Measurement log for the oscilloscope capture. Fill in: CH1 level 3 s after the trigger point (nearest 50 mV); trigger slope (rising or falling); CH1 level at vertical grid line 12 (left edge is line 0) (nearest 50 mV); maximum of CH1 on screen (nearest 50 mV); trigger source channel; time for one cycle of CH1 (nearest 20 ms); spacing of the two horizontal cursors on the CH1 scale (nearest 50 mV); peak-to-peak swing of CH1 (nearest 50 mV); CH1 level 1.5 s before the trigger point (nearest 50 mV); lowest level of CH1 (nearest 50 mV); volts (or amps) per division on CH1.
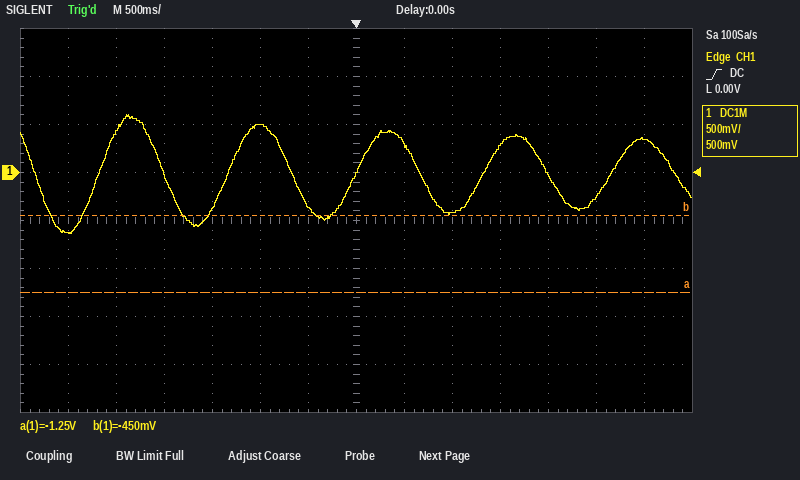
350 mV
rising
-250 mV
600 mV
CH1
1.34 s
800 mV
1.25 V
-400 mV
-650 mV
500 mV
